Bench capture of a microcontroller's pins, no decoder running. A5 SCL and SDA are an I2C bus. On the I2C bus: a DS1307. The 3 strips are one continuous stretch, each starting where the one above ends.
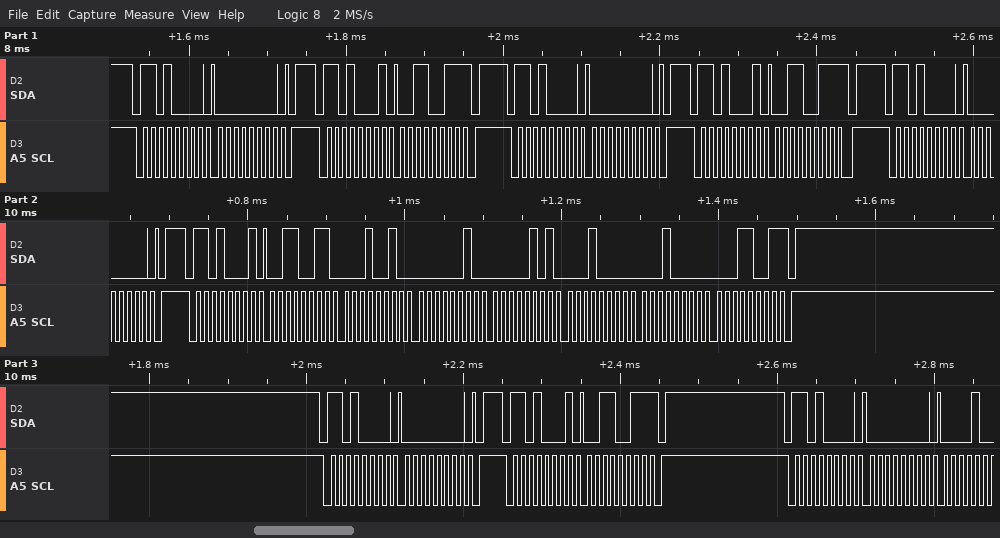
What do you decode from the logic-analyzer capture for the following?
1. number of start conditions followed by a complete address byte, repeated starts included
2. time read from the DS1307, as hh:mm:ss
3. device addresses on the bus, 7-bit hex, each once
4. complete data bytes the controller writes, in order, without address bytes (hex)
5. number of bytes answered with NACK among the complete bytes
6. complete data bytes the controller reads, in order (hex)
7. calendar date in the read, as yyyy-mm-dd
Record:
9
02:12:33
0x68
00 00 00 00 00
4
33 33 33 12 02 05 10 10 19 33
2019-10-10
